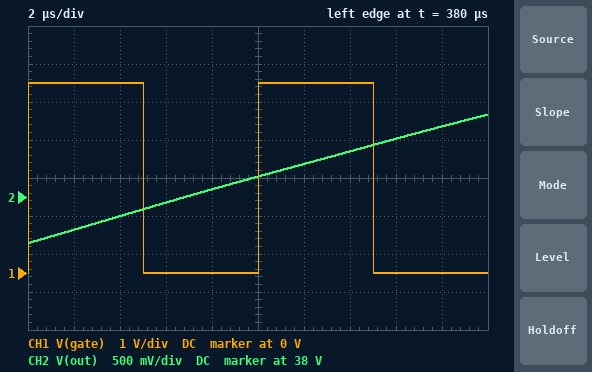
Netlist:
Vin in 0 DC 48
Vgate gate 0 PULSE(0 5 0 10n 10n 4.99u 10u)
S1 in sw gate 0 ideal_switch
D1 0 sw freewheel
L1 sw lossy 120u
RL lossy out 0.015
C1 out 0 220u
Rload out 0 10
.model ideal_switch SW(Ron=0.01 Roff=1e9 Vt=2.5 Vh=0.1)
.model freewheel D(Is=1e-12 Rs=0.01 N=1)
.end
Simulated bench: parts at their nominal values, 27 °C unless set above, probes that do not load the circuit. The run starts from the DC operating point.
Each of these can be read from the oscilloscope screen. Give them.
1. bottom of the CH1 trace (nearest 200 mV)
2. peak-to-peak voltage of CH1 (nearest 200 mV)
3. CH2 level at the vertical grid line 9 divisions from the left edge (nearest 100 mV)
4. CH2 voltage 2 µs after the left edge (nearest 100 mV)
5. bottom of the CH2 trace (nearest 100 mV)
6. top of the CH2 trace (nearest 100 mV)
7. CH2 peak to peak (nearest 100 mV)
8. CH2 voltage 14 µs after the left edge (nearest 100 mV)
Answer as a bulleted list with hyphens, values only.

- 0 V
- 5.0 V
- 38.9 V
- 37.6 V
- 37.4 V
- 39.1 V
- 1.7 V
- 38.6 V
